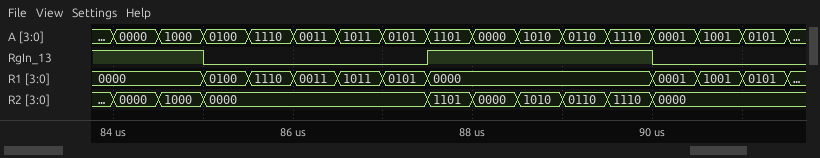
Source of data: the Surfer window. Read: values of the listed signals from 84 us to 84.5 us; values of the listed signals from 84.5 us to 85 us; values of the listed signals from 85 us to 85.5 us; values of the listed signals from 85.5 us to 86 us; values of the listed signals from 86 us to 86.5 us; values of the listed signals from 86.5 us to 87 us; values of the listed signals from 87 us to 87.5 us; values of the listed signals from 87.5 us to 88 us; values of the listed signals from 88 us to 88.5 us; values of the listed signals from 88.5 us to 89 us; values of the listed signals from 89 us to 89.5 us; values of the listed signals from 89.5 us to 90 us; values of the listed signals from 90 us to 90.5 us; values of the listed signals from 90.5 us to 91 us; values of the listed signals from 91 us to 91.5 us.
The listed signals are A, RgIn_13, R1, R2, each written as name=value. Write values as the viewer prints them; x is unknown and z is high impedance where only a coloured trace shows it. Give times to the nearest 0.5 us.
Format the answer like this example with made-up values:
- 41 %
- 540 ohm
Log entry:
- A=0000, RgIn_13=1, R1=0000, R2=0000
- A=1000, RgIn_13=1, R1=0000, R2=1000
- A=0100, RgIn_13=0, R1=0100, R2=0000
- A=1110, RgIn_13=0, R1=1110, R2=0000
- A=0011, RgIn_13=0, R1=0011, R2=0000
- A=1011, RgIn_13=0, R1=1011, R2=0000
- A=0101, RgIn_13=0, R1=0101, R2=0000
- A=1101, RgIn_13=1, R1=0000, R2=1101
- A=0000, RgIn_13=1, R1=0000, R2=0000
- A=1010, RgIn_13=1, R1=0000, R2=1010
- A=0110, RgIn_13=1, R1=0000, R2=0110
- A=1110, RgIn_13=1, R1=0000, R2=1110
- A=0001, RgIn_13=0, R1=0001, R2=0000
- A=1001, RgIn_13=0, R1=1001, R2=0000
- A=0101, RgIn_13=0, R1=0101, R2=0000
